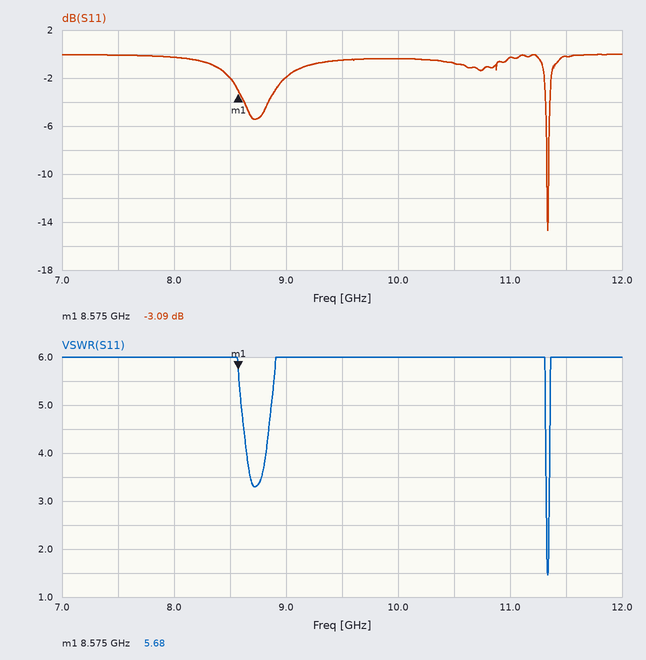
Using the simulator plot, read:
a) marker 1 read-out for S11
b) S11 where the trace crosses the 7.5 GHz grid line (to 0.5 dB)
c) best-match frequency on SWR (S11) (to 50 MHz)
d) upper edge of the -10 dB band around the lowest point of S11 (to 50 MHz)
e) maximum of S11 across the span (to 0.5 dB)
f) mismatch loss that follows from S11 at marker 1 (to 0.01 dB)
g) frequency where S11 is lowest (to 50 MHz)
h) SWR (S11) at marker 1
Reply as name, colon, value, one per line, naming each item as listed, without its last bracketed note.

marker 1 read-out for S11: -3.09 dB
S11 where the trace crosses the 7.5 GHz grid line: 0.0 dB
best-match frequency on SWR (S11): 11.35 GHz
upper edge of the -10 dB band around the lowest point of S11: 11.35 GHz
maximum of S11 across the span: 0.0 dB
mismatch loss that follows from S11 at marker 1: 2.93 dB
frequency where S11 is lowest: 11.35 GHz
SWR (S11) at marker 1: 5.68
